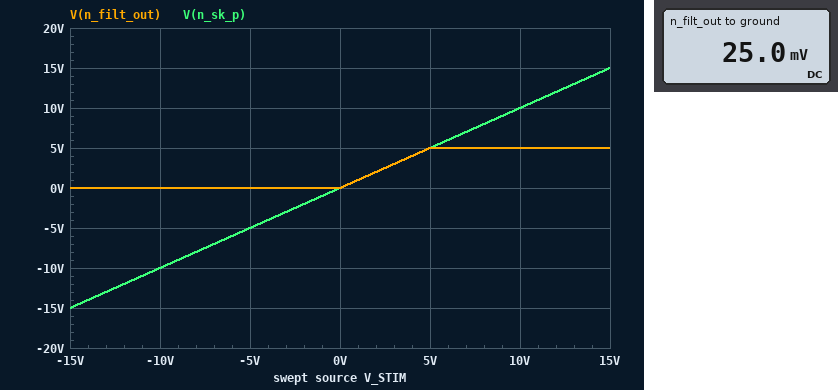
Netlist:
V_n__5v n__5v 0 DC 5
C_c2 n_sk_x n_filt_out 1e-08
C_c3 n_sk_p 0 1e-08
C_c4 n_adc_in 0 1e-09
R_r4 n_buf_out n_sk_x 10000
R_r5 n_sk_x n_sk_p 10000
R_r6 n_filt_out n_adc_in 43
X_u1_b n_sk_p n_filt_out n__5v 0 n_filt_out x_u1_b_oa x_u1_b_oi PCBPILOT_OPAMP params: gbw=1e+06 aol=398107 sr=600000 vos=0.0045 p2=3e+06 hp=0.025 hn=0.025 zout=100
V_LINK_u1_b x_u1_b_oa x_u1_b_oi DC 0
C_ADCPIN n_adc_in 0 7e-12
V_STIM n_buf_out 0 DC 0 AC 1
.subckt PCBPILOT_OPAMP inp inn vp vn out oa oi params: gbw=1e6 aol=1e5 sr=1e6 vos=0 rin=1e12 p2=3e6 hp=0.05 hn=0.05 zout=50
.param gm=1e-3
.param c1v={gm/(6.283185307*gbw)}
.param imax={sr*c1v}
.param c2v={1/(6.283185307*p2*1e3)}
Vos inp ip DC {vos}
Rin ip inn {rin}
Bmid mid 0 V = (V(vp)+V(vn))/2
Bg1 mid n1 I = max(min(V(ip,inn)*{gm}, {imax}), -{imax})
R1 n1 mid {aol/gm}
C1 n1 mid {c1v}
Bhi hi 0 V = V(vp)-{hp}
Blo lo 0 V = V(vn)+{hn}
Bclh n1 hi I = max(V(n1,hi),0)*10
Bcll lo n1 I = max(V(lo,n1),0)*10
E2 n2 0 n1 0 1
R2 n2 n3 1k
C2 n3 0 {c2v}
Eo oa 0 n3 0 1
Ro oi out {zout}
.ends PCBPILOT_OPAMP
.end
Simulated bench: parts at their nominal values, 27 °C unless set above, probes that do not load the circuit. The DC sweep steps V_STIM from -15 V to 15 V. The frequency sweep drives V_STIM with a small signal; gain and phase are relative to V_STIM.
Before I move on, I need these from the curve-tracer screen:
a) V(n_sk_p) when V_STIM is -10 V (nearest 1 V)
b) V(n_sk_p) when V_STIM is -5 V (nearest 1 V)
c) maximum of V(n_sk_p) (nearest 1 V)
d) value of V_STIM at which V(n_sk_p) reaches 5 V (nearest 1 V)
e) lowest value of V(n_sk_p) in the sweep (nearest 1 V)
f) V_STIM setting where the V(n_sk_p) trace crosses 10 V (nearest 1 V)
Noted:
-10 V
-5 V
15 V
5 V
-15 V
10 V
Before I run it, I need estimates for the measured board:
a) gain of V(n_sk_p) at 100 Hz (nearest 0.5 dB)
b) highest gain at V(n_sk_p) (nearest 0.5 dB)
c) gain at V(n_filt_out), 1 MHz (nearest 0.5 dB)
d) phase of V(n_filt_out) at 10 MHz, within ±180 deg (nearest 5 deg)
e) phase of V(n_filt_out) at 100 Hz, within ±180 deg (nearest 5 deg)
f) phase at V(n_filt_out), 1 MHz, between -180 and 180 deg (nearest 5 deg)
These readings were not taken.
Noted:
0 dB
0 dB
-42.5 dB
-15 deg
75 deg
-25 deg
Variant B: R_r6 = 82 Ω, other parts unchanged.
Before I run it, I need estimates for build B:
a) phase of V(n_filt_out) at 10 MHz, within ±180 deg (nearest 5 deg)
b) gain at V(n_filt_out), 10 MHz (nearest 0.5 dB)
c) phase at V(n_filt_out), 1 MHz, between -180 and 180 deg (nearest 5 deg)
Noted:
-5 deg
-47.0 dB
-20 deg
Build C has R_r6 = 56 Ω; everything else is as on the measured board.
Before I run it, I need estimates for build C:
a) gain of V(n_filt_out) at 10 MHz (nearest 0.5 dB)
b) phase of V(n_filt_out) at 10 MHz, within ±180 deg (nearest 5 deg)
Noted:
-48.5 dB
-10 deg
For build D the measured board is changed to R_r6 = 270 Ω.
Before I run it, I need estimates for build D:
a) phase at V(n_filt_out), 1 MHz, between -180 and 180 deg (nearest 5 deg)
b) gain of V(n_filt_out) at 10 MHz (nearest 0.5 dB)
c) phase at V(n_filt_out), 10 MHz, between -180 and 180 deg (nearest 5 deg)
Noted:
-5 deg
-43.0 dB
0 deg
